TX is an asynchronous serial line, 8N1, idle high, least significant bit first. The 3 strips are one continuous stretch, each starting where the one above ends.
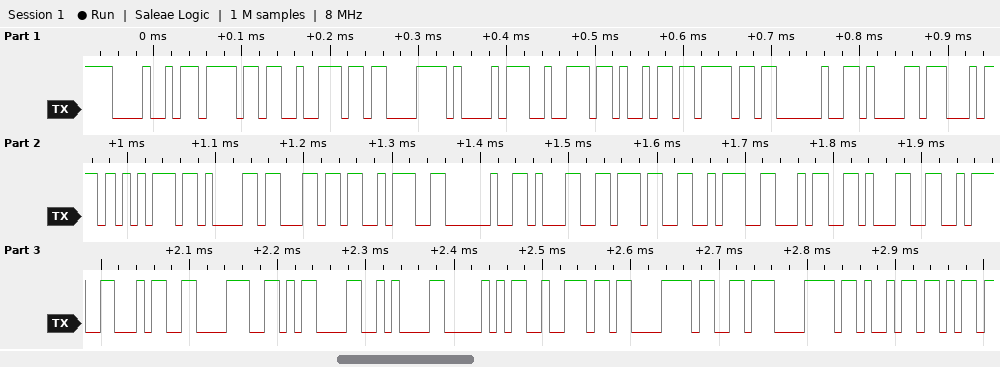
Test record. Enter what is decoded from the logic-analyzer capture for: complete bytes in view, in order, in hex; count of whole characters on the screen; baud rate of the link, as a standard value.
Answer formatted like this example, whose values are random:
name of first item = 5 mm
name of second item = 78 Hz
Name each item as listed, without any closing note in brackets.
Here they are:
complete bytes in view, in order, in hex = 48 6F 72 C3 A1 72 69 6F 20 61 74 75 61 6C 3A 20 31 37 3A 34 31 3A 34 38 0D 0A 50 72 C3 B3 78 69
count of whole characters on the screen = 32
baud rate of the link, as a standard value = 115200 baud
